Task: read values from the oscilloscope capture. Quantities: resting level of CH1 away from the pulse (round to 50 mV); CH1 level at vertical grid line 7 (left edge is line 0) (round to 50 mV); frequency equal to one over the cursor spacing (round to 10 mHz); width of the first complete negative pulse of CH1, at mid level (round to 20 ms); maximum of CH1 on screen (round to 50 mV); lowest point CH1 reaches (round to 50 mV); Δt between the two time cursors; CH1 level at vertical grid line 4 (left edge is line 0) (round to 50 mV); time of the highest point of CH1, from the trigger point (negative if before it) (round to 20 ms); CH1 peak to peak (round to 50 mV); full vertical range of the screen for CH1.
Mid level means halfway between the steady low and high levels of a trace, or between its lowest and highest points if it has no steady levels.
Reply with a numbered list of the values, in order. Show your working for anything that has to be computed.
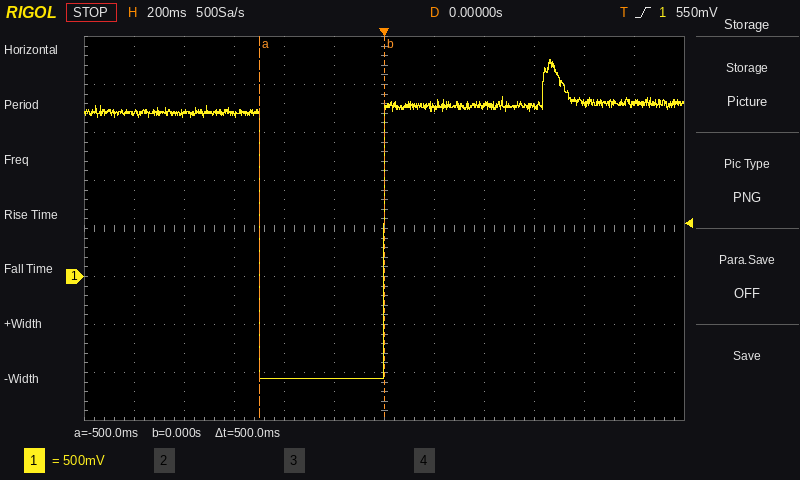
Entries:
1. 1.75 V
2. 1.75 V
3. 1 / 500 ms ≈ 2.00 Hz
4. 500 ms
5. 2.25 V
6. -1.05 V
7. 500 ms
8. -1.05 V
9. +660 ms
10. 2.25 V − (-1.05 V) = 3.30 V
11. 4 V
